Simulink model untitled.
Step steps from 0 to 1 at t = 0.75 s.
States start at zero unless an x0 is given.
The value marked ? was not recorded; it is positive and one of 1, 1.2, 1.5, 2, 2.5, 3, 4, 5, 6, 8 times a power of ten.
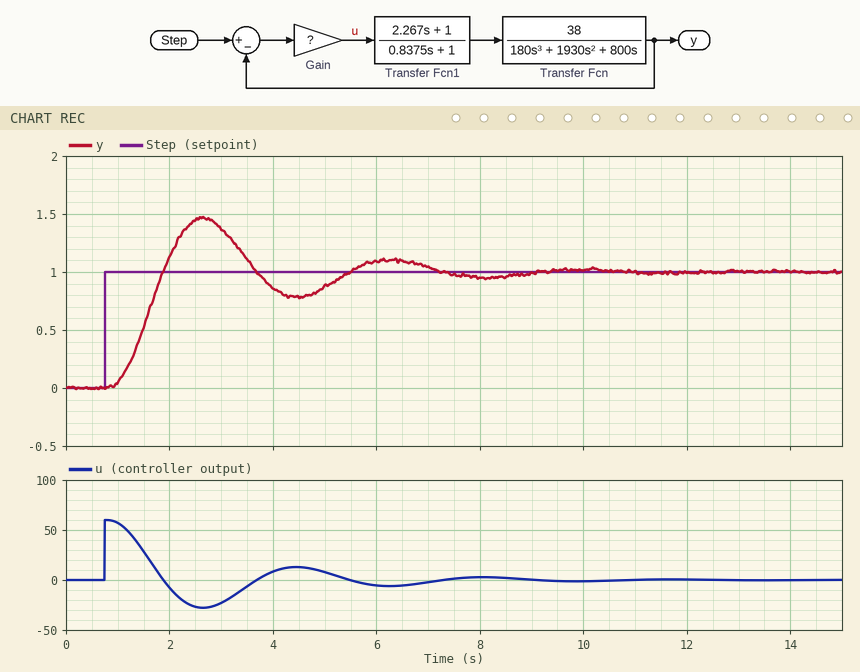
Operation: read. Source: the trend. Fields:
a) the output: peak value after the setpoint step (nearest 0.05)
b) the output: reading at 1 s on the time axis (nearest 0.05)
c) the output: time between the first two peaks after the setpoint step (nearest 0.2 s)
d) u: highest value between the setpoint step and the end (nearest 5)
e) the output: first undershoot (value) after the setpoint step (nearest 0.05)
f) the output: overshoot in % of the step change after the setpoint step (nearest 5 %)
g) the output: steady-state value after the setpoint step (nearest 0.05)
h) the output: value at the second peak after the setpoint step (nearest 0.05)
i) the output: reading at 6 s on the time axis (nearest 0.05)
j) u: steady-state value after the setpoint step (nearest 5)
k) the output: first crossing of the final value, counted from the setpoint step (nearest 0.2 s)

1.45
0.05
3.6 s
60
0.80
45 %
1.00
1.10
1.10
0
1.2 s
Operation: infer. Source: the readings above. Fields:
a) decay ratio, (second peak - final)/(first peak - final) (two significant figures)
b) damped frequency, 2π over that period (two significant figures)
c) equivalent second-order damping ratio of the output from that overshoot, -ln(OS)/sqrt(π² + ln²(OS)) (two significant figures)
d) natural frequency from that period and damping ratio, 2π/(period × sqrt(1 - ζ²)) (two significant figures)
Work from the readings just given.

0.22
1.7 rad/s
0.25
1.8 rad/s
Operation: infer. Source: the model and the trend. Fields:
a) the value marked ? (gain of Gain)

60
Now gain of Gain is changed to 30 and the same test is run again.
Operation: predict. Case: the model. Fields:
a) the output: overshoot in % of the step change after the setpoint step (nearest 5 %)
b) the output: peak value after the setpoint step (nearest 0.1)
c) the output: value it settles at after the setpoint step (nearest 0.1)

25 %
1.3
1.0
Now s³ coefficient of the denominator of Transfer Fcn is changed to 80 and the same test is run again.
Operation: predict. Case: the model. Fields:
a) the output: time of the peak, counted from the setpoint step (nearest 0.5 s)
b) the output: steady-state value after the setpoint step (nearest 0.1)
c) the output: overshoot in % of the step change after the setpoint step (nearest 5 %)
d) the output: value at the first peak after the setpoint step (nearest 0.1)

2.0 s
1.0
40 %
1.4
